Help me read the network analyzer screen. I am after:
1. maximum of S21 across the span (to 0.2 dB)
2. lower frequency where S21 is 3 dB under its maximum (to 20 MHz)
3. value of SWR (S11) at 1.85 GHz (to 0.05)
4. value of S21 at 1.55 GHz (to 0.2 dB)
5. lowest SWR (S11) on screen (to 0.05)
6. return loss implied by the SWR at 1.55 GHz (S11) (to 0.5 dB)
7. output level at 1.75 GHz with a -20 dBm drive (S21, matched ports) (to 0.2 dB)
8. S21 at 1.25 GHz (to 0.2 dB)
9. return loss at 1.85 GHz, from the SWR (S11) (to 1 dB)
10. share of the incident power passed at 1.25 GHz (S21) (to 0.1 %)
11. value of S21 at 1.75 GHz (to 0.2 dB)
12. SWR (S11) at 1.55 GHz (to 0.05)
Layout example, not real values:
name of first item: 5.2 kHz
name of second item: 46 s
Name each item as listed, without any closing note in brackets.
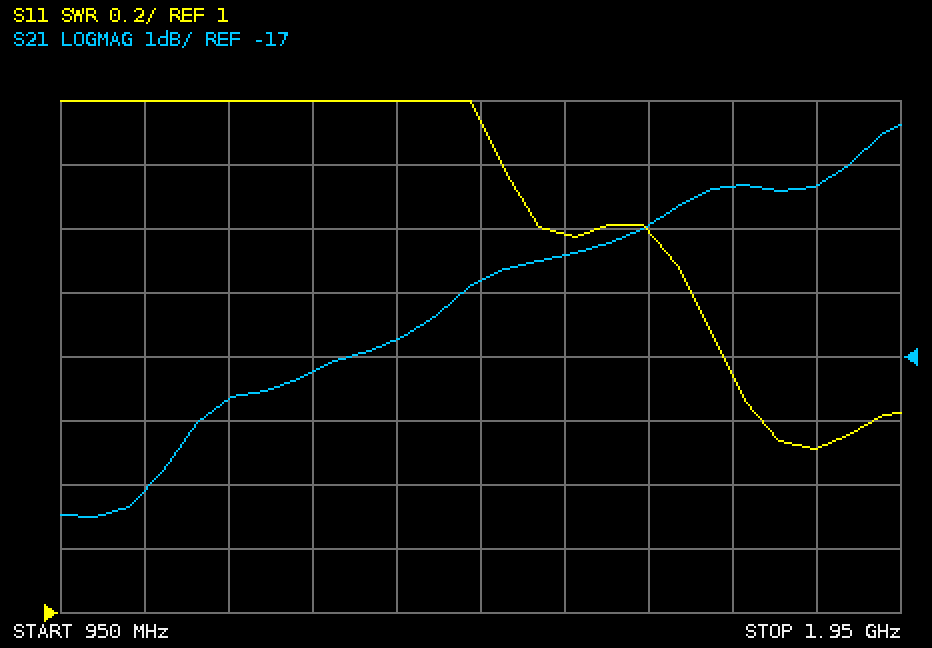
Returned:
maximum of S21 across the span: -13.4 dB
lower frequency where S21 is 3 dB under its maximum: 1.40 GHz
value of SWR (S11) at 1.85 GHz: 1.50
value of S21 at 1.55 GHz: -15.4 dB
lowest SWR (S11) on screen: 1.50
return loss implied by the SWR at 1.55 GHz (S11): 8.5 dB
output level at 1.75 GHz with a -20 dBm drive (S21, matched ports): -34.4 dBm
S21 at 1.25 GHz: -17.2 dB
return loss at 1.85 GHz, from the SWR (S11): 14 dB
share of the incident power passed at 1.25 GHz (S21): 1.9 %
value of S21 at 1.75 GHz: -14.4 dB
SWR (S11) at 1.55 GHz: 2.20
